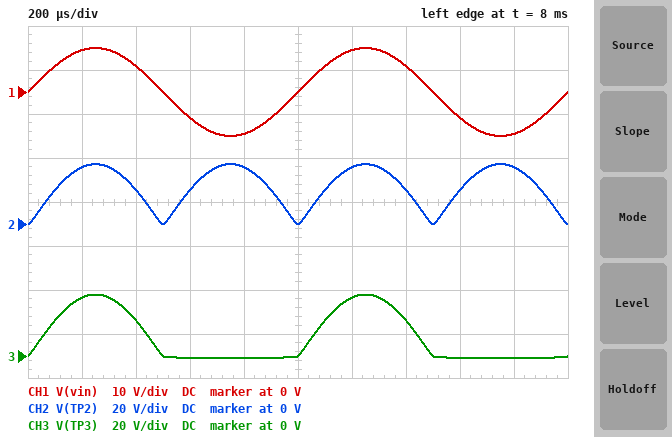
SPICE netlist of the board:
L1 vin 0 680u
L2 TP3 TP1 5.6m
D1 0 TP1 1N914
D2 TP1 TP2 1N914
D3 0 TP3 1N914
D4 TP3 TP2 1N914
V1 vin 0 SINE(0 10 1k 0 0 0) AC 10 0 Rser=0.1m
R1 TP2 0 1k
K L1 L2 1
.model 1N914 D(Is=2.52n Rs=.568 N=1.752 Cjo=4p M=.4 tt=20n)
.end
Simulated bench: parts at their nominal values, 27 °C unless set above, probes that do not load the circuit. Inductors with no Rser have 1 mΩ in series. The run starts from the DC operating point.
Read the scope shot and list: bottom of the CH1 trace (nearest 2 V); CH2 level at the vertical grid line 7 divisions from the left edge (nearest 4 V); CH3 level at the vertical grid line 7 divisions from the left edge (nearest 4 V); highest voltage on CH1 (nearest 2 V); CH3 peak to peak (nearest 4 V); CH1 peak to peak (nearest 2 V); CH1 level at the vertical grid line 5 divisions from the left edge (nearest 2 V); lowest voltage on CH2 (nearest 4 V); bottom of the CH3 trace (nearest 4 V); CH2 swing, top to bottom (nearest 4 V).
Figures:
-10 V
16 V
16 V
10 V
28 V
20 V
0 V
0 V
0 V
28 V
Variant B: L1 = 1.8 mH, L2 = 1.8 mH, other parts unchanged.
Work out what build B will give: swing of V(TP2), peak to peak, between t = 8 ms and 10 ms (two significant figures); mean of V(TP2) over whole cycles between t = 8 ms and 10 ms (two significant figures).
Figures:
8.6 V
5.1 V
